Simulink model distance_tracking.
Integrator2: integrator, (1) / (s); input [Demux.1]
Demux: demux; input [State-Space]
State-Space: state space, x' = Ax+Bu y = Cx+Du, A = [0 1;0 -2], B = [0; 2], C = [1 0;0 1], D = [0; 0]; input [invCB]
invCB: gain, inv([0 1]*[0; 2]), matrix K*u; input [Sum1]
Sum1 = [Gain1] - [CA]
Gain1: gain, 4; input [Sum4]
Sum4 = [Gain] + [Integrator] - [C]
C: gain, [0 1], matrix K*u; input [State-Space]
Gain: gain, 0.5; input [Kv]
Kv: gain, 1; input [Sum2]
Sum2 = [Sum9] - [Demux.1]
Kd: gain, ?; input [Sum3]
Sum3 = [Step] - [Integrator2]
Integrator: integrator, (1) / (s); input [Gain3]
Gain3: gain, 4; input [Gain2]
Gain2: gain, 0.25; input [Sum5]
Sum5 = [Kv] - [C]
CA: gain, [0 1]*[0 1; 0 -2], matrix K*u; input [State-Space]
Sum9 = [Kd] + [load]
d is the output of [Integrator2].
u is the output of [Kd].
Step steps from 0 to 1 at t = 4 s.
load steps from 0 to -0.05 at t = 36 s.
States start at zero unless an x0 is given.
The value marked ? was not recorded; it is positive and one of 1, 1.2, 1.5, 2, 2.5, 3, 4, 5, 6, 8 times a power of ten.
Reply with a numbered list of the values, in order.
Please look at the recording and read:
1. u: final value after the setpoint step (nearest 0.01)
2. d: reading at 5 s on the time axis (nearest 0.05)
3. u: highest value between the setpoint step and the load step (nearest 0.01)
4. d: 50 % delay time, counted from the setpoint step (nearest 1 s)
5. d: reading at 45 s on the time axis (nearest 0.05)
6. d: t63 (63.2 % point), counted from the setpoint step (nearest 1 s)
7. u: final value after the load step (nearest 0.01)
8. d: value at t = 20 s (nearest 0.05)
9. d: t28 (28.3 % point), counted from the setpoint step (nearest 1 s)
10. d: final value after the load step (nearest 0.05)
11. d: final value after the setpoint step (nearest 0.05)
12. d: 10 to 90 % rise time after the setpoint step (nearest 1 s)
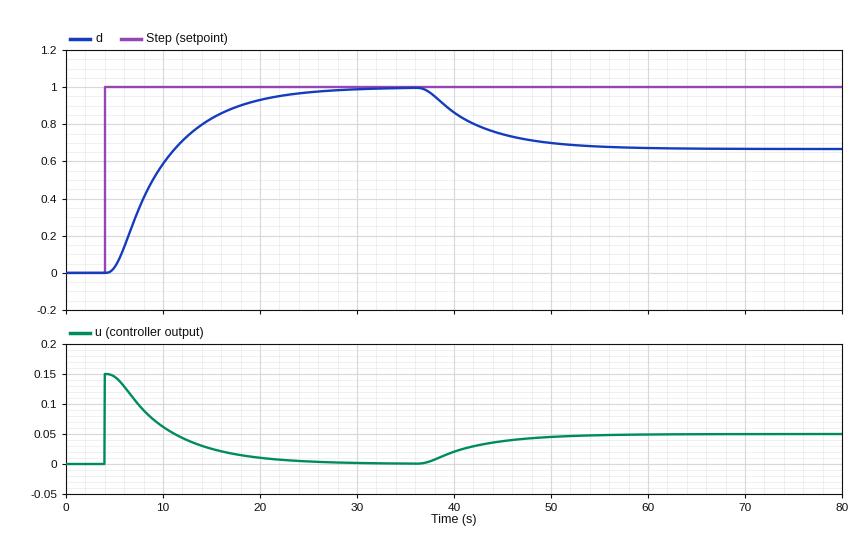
1. 0.00
2. 0.05
3. 0.15
4. 5 s
5. 0.75
6. 7 s
7. 0.05
8. 0.95
9. 3 s
10. 0.65
11. 1.00
12. 12 s
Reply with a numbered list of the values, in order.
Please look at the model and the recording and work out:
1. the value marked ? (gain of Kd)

1. 0.15
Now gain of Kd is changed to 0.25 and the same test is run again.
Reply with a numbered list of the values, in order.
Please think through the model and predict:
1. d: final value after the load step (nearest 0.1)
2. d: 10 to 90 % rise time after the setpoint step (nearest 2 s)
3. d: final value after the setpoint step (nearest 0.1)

1. 0.8
2. 6 s
3. 1.0
